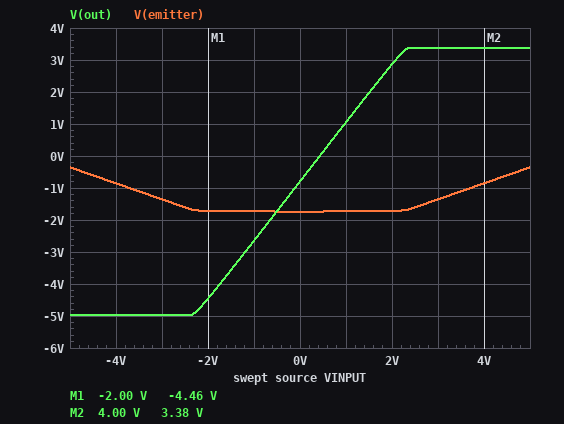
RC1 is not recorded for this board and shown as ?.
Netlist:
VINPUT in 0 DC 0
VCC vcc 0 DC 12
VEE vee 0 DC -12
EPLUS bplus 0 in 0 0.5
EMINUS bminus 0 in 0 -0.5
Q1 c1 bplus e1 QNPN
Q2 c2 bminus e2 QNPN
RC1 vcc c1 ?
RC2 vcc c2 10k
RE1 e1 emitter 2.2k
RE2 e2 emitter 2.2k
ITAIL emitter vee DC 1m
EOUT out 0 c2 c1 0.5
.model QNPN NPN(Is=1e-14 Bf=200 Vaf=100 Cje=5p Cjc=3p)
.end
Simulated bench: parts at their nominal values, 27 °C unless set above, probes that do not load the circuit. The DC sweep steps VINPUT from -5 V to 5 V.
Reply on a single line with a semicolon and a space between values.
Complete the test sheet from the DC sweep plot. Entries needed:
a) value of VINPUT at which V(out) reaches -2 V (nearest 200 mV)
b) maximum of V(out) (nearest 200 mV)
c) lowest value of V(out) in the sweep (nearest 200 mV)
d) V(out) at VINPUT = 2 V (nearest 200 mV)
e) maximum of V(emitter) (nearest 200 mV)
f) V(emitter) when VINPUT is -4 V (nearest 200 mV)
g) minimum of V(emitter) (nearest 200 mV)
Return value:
-600 mV; 3.4 V; -5.0 V; 2.8 V; -400 mV; -800 mV; -1.8 V
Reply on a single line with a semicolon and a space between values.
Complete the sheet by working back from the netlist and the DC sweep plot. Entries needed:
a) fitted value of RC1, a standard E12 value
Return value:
6.8 kΩ
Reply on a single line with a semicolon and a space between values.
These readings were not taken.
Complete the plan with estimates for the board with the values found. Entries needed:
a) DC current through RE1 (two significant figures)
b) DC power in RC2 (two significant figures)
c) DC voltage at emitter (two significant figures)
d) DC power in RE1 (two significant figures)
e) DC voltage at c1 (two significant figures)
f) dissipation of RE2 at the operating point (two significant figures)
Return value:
500 µA; 2.5 mW; -1.7 V; 550 µW; 8.6 V; 550 µW
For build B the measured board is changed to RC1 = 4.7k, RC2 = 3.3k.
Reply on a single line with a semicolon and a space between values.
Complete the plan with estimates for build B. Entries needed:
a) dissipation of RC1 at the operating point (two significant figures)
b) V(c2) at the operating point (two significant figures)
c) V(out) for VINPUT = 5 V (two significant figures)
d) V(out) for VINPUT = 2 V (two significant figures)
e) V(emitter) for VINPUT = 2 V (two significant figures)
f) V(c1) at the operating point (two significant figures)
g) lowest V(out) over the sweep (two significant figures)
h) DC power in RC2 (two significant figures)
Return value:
1.2 mW; 10 V; 2.3 V; 2.1 V; -1.7 V; 9.7 V; -1.6 V; 820 µW
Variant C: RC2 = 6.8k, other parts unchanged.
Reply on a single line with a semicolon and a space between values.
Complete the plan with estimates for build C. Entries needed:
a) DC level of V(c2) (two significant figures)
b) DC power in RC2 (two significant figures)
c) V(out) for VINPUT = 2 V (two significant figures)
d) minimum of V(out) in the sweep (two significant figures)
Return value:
8.6 V; 1.7 mW; 3.0 V; -3.4 V
